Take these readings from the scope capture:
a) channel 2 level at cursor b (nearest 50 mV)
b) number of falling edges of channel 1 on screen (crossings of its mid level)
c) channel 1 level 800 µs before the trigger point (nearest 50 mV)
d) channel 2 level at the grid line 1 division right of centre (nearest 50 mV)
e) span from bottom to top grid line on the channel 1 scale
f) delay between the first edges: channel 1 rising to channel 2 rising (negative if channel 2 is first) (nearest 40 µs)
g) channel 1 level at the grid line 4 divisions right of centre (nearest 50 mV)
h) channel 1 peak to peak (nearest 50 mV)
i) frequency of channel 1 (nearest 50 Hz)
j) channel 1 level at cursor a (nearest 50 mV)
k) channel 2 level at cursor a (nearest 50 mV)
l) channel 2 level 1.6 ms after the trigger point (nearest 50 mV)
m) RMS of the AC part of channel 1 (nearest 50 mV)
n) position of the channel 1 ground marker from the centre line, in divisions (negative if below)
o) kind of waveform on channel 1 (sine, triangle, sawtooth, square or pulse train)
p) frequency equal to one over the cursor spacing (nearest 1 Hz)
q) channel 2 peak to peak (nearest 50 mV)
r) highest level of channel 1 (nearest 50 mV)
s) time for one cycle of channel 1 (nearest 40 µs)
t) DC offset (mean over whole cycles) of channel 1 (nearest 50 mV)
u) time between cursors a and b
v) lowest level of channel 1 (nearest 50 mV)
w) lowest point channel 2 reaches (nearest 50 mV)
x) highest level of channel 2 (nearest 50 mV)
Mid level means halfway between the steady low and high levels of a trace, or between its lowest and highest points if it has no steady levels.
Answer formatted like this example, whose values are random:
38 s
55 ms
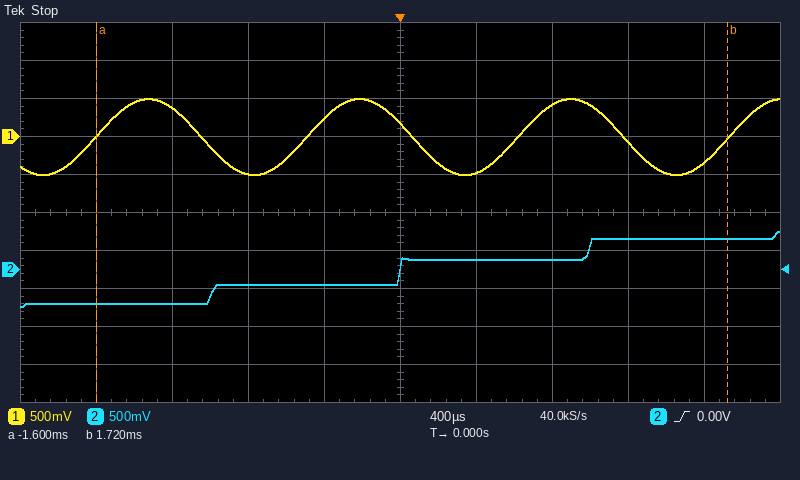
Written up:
400 mV
3
-500 mV
150 mV
5 V
+1.60 ms
-350 mV
1.00 V
900 Hz
0 mV
-450 mV
400 mV
350 mV
+2.0 div
sine
301 Hz
1.00 V
500 mV
1.12 ms
0 mV
3.32 ms
-500 mV
-500 mV
500 mV
